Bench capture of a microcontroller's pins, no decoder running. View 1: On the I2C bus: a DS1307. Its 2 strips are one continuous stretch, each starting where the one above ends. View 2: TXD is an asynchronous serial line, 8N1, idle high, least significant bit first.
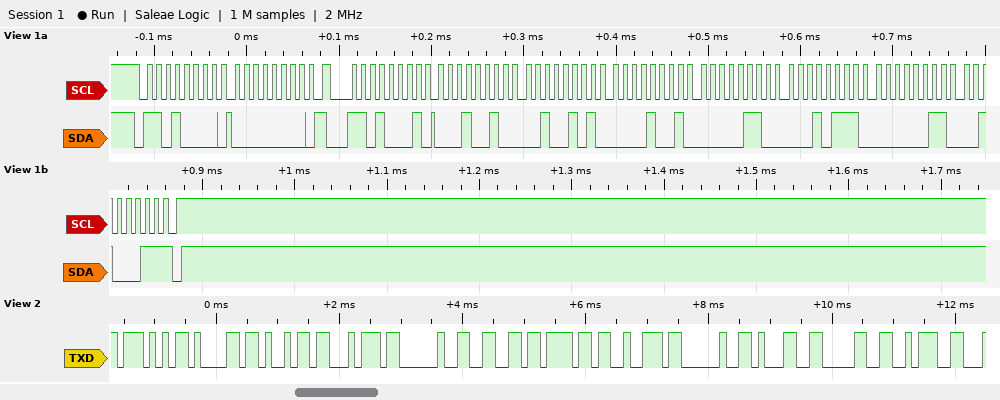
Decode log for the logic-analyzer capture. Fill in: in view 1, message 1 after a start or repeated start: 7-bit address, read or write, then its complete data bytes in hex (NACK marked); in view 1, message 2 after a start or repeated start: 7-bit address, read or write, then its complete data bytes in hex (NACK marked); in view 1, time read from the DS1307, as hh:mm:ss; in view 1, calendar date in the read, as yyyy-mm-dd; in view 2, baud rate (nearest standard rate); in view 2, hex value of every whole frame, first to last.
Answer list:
0x68 write: 00
0x68 read: 12 25 09 06 17 03 23 NACK
09:25:12
2023-03-17
9600 baud
57 61 69 74 20 66 6F 72 20 31 30 3A
